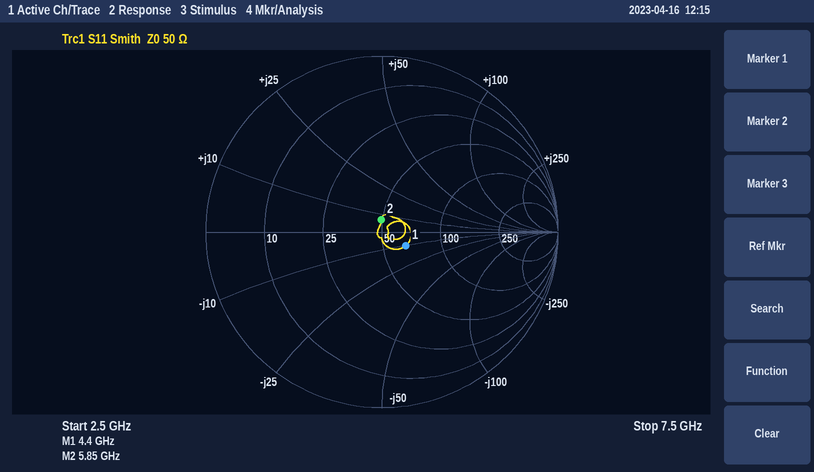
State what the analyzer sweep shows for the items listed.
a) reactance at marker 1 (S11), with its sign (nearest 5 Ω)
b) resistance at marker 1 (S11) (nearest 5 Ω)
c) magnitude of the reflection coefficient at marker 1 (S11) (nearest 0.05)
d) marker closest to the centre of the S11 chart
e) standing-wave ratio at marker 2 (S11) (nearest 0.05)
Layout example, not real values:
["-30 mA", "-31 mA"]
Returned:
["-10 Ω", "65 Ω", "0.15", "marker 2", "1.15"]
